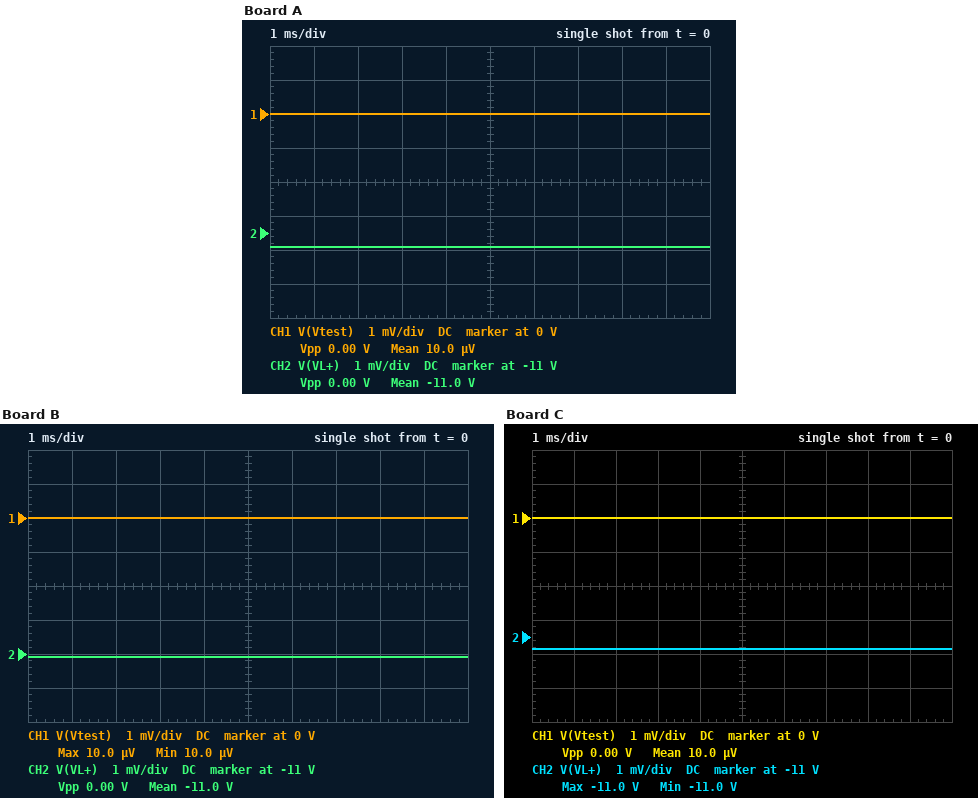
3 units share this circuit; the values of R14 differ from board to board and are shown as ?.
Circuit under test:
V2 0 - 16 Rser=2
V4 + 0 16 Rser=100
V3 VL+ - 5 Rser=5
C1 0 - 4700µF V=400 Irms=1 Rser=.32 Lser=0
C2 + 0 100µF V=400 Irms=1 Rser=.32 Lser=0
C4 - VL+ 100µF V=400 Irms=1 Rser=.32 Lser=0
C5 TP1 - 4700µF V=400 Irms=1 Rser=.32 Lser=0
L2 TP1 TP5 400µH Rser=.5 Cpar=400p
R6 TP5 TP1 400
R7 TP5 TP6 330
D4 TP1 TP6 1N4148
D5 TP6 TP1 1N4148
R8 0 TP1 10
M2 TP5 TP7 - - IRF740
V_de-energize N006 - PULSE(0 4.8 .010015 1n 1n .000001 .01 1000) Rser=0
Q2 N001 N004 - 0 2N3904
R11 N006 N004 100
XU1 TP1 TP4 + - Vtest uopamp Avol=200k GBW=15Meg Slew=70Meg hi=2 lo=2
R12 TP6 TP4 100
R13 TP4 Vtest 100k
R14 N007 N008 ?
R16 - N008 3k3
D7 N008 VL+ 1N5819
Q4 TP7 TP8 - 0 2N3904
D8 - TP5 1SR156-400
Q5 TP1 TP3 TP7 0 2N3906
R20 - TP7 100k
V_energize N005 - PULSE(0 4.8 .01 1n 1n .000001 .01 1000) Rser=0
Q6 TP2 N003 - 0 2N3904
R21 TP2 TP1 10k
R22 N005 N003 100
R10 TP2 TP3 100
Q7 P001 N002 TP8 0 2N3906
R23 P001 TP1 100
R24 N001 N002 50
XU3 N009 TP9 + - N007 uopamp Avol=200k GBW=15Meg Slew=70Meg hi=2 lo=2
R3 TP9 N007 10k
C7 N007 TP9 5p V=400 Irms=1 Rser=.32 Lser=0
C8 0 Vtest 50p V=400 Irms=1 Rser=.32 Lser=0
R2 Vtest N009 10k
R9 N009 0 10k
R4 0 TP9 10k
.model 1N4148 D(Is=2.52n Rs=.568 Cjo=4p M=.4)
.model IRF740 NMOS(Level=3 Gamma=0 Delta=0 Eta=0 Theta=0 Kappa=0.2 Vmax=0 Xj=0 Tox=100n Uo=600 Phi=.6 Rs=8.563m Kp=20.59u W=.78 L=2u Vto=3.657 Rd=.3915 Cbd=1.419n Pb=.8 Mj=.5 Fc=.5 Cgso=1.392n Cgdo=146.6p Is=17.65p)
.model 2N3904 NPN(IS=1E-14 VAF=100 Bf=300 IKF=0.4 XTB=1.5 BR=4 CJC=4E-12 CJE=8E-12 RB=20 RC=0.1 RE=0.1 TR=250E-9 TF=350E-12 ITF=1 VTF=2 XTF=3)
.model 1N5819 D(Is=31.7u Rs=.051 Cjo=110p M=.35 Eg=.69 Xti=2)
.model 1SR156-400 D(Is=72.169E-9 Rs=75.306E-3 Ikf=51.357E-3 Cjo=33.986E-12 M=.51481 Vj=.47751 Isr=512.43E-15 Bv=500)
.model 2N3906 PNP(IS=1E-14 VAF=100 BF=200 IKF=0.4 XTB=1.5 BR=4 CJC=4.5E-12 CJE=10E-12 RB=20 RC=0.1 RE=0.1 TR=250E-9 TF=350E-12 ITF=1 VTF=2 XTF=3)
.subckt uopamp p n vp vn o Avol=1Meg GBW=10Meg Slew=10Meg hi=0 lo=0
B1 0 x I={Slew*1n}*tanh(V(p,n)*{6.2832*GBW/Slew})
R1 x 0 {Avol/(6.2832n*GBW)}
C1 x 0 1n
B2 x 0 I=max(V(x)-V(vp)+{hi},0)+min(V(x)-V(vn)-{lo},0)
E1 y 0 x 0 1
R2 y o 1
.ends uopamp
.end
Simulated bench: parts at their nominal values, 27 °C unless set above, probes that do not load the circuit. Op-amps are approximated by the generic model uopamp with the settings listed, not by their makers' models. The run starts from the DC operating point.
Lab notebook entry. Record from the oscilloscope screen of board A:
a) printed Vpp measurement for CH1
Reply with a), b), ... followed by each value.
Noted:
a) 0.00 V
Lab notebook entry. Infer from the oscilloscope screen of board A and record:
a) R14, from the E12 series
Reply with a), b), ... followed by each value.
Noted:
a) 15 kΩ
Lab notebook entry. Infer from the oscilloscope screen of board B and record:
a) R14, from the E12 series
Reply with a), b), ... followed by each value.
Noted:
a) 12 kΩ
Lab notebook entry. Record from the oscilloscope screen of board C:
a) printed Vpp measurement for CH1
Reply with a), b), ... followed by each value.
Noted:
a) 0.00 V
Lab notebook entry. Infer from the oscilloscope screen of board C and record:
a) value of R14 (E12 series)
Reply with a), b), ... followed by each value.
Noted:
a) 6.8 kΩ
